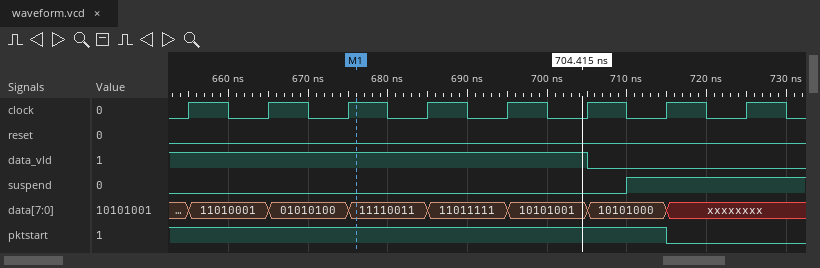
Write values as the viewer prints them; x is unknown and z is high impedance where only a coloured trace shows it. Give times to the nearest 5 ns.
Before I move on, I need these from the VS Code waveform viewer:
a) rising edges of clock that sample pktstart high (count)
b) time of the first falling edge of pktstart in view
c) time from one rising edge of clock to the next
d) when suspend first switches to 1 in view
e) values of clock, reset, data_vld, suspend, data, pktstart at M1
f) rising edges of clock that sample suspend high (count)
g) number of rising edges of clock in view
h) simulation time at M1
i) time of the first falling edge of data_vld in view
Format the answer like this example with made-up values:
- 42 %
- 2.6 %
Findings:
- 7
- 715 ns
- 10 ns
- 710 ns
- clock=1, reset=0, data_vld=1, suspend=0, data=11110011, pktstart=1
- 2
- 8
- 675 ns
- 705 ns
